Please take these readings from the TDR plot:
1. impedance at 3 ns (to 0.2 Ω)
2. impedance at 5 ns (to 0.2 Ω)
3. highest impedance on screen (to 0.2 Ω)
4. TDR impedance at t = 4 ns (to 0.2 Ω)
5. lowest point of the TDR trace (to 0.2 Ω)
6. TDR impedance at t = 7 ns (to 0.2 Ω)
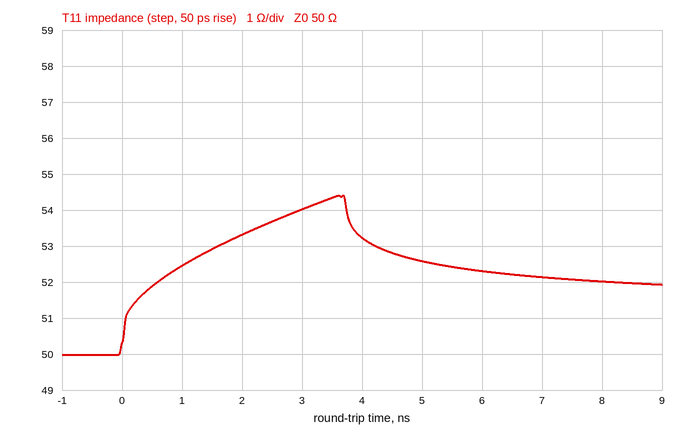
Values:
54.0 Ω
52.6 Ω
54.4 Ω
53.2 Ω
50.0 Ω
52.2 Ω
